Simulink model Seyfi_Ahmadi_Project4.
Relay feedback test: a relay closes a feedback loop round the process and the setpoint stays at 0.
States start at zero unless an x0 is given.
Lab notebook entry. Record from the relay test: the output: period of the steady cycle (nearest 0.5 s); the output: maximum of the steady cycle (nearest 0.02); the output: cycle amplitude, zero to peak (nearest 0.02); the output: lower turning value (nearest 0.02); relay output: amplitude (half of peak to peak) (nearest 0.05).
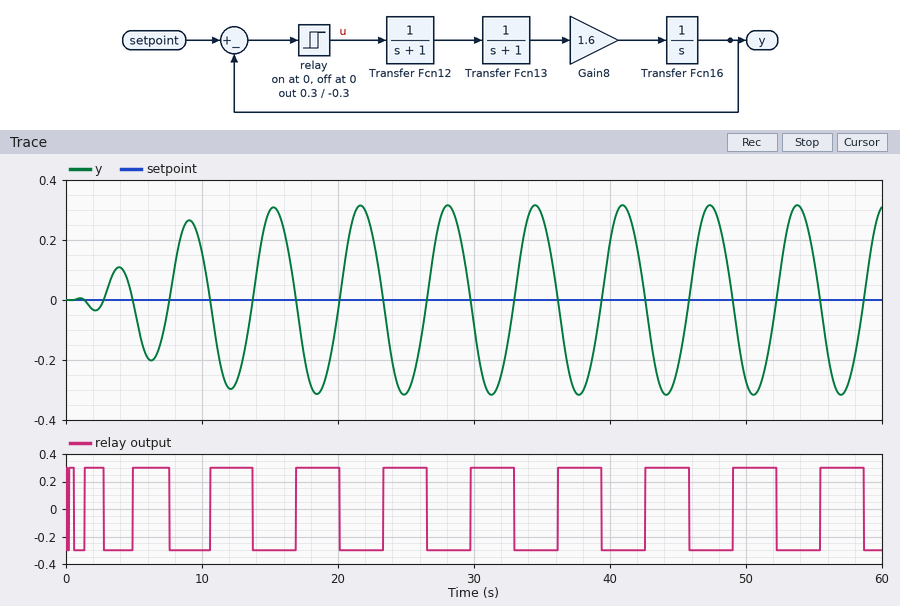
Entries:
6.5 s
0.32
0.32
-0.32
0.30
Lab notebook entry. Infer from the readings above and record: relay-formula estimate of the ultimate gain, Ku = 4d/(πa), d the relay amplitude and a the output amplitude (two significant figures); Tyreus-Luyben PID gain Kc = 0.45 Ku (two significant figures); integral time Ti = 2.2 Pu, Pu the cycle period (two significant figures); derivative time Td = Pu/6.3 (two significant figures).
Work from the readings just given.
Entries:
1.2
0.54
14 s
1.0 s
